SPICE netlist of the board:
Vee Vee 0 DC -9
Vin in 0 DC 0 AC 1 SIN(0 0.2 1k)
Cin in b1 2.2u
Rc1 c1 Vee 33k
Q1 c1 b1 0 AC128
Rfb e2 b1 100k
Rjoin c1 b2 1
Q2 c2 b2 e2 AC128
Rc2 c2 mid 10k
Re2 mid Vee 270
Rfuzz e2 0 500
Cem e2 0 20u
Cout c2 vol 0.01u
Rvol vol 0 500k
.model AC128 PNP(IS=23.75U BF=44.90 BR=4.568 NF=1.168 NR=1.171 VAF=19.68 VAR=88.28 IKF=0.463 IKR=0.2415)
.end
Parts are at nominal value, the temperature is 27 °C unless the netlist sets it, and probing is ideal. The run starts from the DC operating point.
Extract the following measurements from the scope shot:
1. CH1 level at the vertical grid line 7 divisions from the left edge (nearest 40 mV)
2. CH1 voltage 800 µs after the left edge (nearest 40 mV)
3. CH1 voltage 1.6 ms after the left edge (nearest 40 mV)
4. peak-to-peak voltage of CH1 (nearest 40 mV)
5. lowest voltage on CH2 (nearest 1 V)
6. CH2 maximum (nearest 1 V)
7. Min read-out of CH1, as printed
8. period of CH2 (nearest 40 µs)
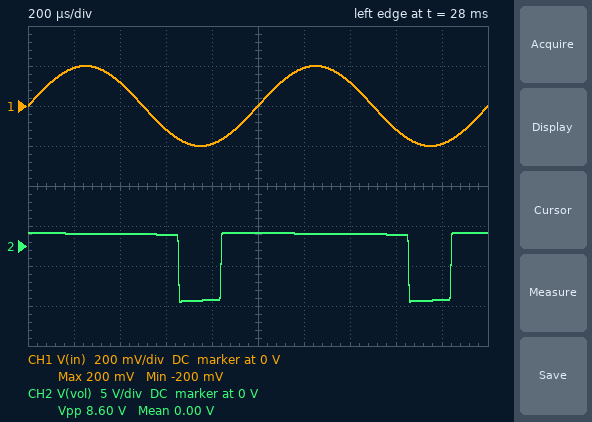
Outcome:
120 mV
-200 mV
-120 mV
400 mV
-7 V
2 V
-200 mV
1.00 ms
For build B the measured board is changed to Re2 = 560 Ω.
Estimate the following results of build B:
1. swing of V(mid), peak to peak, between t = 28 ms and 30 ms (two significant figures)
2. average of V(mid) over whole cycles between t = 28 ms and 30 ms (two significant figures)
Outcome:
440 mV
-8.6 V
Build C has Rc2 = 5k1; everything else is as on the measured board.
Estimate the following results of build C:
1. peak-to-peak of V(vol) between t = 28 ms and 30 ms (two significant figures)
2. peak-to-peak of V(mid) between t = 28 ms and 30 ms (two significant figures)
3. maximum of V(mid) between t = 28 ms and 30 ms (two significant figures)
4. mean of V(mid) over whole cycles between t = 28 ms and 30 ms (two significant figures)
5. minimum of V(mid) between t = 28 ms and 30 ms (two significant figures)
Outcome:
8.4 V
410 mV
-8.6 V
-8.7 V
-9.0 V
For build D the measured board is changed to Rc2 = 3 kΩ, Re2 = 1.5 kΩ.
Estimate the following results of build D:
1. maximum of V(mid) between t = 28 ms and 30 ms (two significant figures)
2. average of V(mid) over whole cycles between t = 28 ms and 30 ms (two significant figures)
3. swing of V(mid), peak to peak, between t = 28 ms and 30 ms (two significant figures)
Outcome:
-6.3 V
-6.8 V
2.7 V
